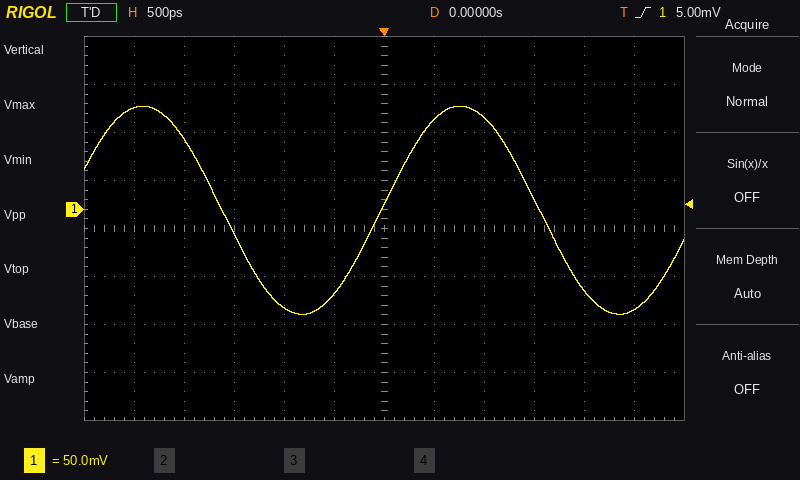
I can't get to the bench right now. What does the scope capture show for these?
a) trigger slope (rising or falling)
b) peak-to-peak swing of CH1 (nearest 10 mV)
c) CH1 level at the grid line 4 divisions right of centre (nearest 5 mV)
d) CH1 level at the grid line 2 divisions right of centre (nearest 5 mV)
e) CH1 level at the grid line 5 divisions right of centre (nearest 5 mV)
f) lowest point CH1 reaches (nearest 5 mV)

rising
220 mV
-85 mV
95 mV
-105 mV
-110 mV
